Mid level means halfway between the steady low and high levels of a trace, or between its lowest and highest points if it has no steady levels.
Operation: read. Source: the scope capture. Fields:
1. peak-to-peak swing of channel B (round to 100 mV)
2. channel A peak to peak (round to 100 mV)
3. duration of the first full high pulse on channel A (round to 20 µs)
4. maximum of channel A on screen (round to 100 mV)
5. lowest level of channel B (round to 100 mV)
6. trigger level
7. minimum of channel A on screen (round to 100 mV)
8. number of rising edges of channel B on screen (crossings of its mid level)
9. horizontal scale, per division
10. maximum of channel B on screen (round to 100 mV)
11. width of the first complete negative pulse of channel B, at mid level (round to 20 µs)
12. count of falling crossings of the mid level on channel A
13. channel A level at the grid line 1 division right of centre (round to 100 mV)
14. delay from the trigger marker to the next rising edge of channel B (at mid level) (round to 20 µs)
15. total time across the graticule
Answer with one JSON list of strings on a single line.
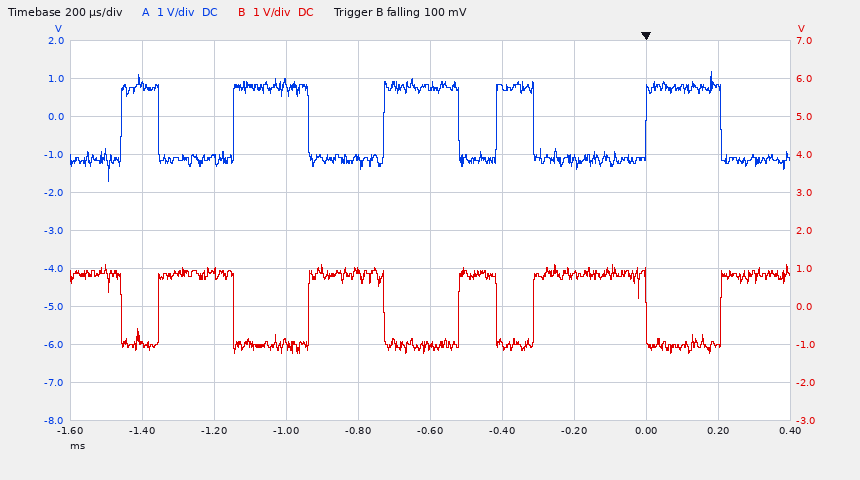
["2.3 V", "2.9 V", "100 µs", "1.2 V", "-1.2 V", "100 mV", "-1.7 V", "5", "200 µs", "1.1 V", "100 µs", "5", "800 mV", "200 µs", "2 ms"]
